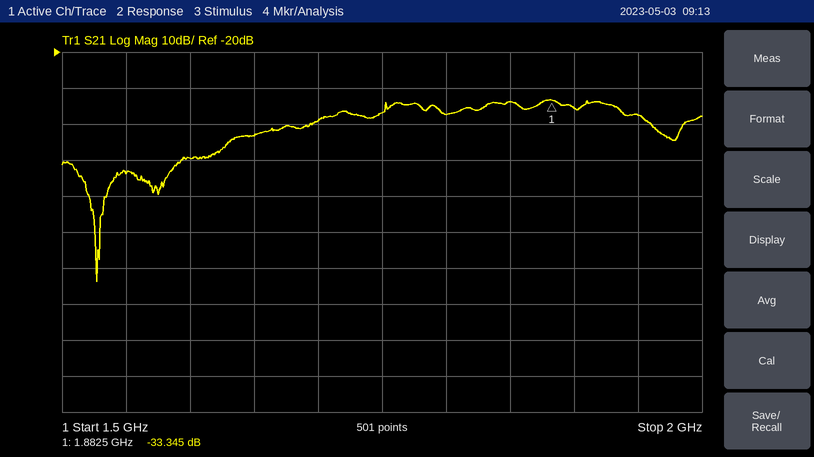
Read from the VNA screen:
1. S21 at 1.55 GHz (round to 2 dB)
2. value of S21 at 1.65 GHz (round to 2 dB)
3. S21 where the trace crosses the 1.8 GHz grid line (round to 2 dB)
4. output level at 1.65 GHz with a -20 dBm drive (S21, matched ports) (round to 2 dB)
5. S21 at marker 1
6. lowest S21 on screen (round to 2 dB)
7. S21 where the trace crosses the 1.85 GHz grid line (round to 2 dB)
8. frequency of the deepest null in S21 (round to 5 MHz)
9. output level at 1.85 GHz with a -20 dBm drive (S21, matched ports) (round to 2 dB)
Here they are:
-54 dB
-44 dB
-38 dB
-64 dBm
-33.345 dB
-84 dB
-34 dB
1.525 GHz
-54 dBm
